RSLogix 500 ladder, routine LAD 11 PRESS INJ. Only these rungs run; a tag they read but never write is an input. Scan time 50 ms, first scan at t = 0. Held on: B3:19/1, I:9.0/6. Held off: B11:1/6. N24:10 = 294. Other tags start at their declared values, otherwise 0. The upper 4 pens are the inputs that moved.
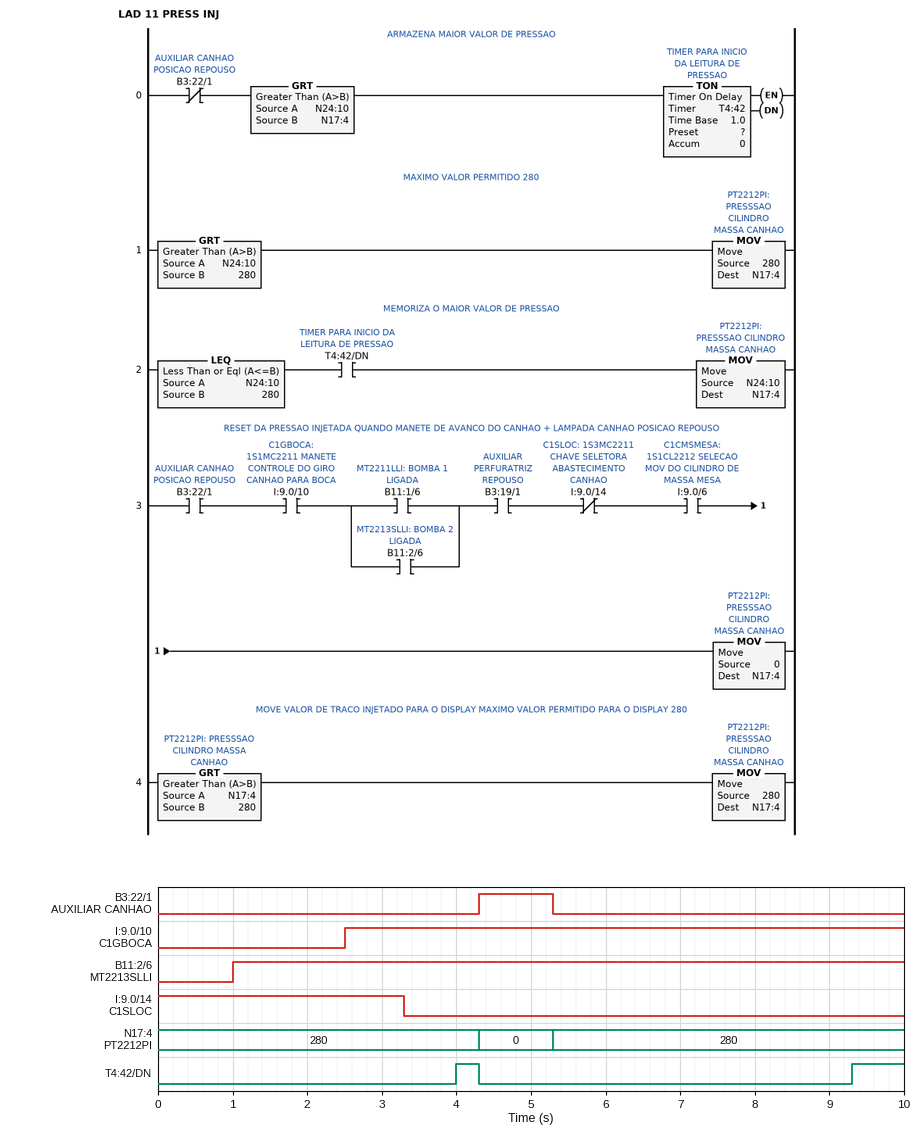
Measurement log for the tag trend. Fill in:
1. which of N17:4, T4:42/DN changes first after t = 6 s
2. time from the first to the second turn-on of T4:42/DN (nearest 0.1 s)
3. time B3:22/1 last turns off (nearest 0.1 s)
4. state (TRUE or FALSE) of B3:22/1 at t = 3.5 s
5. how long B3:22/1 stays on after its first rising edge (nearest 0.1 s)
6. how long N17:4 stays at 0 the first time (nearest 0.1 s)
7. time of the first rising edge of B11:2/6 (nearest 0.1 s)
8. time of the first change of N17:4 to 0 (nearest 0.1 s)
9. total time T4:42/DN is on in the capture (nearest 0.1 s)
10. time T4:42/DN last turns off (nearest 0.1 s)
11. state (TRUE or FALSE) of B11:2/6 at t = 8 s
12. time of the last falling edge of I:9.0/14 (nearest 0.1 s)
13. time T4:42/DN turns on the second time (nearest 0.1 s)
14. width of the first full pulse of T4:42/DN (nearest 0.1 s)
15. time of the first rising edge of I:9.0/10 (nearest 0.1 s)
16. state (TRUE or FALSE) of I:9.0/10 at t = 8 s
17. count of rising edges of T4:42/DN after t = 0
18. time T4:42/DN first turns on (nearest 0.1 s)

T4:42/DN
5.3 s
5.3 s
FALSE
1.0 s
1.0 s
1.0 s
4.3 s
1.0 s
4.3 s
TRUE
3.3 s
9.3 s
0.3 s
2.5 s
TRUE
2
4.0 s
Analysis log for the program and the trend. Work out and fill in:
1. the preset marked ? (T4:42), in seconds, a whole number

4 s
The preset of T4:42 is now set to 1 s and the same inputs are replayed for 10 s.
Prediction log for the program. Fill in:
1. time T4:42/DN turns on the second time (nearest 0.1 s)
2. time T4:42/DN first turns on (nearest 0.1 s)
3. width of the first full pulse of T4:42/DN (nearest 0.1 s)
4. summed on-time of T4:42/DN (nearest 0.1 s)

6.3 s
1.0 s
3.3 s
7.0 s
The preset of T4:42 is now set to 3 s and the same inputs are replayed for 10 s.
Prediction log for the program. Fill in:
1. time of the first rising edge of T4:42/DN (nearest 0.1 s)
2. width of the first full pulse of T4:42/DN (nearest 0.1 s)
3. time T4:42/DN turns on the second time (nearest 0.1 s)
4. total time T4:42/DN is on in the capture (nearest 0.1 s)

3.0 s
1.3 s
8.3 s
3.0 s
